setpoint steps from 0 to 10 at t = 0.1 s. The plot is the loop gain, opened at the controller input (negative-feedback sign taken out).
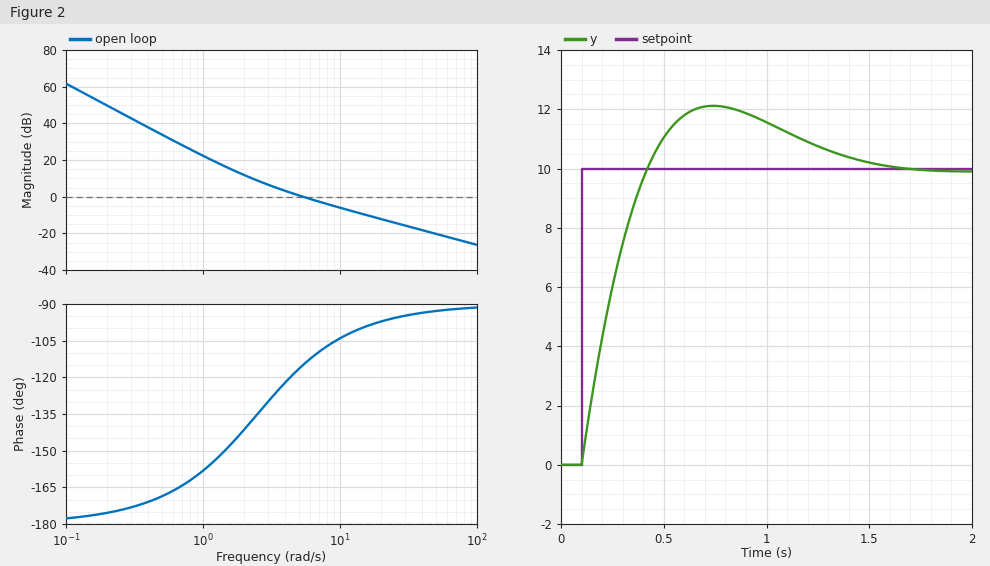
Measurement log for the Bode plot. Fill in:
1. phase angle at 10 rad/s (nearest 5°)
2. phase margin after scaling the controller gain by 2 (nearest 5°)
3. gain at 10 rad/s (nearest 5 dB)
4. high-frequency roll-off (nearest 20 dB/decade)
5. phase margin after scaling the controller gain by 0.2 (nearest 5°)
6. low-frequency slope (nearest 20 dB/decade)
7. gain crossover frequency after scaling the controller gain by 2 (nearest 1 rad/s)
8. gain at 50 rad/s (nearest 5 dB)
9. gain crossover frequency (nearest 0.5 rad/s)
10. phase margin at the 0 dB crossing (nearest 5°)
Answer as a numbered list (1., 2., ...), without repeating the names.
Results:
1. -105°
2. 75°
3. -5 dB
4. -20 dB/decade
5. 35°
6. -40 dB/decade
7. 10 rad/s
8. -20 dB
9. 5.5 rad/s
10. 65°
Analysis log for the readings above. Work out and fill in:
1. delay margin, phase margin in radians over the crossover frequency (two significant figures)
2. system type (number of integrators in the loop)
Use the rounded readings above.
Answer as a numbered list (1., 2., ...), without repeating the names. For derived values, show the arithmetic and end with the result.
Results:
1. 65 × π / 180 / 5.5 = 0.21 s
2. 2
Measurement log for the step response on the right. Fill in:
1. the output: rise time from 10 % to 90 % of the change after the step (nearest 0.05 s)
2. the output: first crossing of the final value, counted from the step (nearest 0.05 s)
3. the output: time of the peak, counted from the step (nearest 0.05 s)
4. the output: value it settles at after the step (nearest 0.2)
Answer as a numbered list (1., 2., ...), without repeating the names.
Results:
1. 0.25 s
2. 0.30 s
3. 0.65 s
4. 10.0
